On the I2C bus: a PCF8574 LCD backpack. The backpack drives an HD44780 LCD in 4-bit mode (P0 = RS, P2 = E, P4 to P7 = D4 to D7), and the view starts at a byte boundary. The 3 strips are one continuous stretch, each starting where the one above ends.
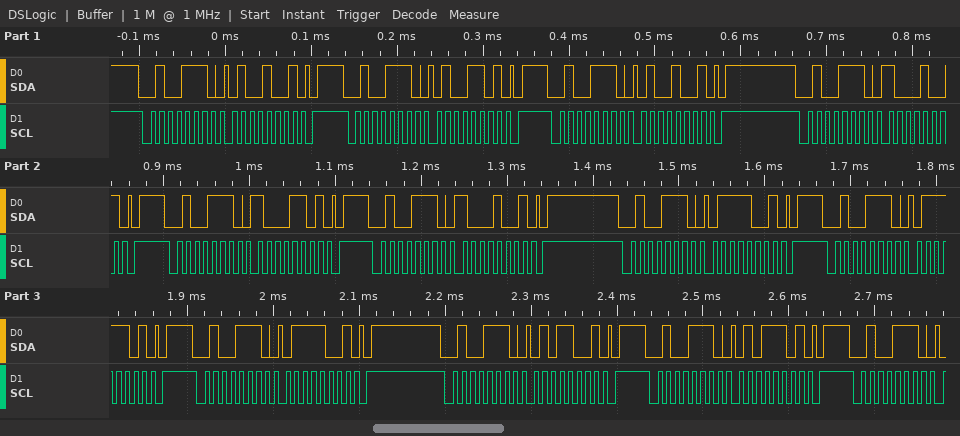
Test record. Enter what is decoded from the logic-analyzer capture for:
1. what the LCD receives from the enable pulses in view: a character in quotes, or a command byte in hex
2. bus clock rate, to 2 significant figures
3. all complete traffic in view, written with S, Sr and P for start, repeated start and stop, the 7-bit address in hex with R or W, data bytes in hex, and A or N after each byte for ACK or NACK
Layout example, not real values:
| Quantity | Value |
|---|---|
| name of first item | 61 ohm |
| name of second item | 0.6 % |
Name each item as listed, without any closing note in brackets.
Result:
| Quantity | Value |
|---|---|
| what the LCD receives from the enable pulses in view: a character in quotes, or a command byte in hex | 'H' |
| bus clock rate, to 2 significant figures | 100 kHz |
| all complete traffic in view, written with S, Sr and P for start, repeated start and stop, the 7-bit address in hex with R or W, data bytes in hex, and A or N after each byte for ACK or NACK | S 27W A 49 A P S 27W A 4D A P S 27W A 49 A P S 27W A 89 A P S 27W A 8D A P S 27W A 89 A P S 27W A 79 A P S 27W A 7D A P S 27W A 79 A P S 27W A 59 A P S 27W A 5D A P S 27W A |
